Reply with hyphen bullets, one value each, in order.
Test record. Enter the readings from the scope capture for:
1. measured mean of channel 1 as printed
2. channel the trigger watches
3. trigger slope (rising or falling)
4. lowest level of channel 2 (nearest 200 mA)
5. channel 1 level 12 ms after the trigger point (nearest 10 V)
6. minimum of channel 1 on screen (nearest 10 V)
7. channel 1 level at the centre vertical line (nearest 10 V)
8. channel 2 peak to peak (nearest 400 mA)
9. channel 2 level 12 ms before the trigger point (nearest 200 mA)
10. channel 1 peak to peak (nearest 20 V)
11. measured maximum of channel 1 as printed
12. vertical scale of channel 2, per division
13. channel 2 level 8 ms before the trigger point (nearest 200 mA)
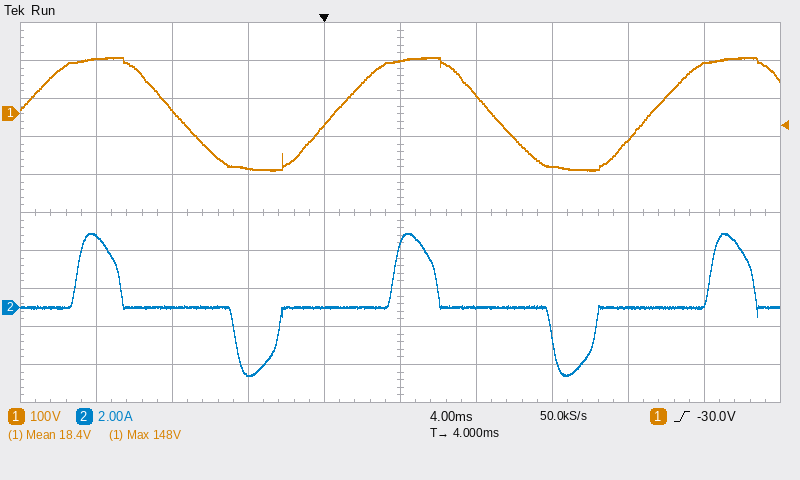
- 18.4 V
- channel 1
- rising
- -3.6 A
- -140 V
- -150 V
- 140 V
- 7.6 A
- 3.8 A
- 300 V
- 148 V
- 2 A
- 0.0 A
